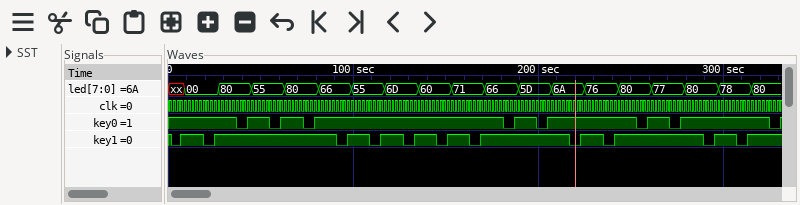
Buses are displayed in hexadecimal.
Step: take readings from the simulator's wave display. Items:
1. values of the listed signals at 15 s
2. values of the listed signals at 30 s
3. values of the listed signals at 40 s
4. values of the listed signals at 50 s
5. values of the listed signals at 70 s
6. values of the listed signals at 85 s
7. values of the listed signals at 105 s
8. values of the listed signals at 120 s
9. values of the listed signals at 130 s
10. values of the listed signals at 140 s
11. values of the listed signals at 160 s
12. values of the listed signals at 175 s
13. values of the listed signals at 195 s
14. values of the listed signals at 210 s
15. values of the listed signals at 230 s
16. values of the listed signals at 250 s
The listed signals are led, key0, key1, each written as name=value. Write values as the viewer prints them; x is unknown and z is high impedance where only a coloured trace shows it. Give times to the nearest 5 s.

led=00, key0=1, key1=1
led=80, key0=1, key1=1
led=80, key0=0, key1=1
led=55, key0=1, key1=1
led=80, key0=1, key1=1
led=66, key0=1, key1=1
led=55, key0=1, key1=1
led=6D, key0=1, key1=1
led=6D, key0=1, key1=0
led=60, key0=1, key1=1
led=71, key0=1, key1=1
led=66, key0=1, key1=1
led=5D, key0=1, key1=1
led=6A, key0=1, key1=1
led=76, key0=1, key1=1
led=80, key0=1, key1=1
